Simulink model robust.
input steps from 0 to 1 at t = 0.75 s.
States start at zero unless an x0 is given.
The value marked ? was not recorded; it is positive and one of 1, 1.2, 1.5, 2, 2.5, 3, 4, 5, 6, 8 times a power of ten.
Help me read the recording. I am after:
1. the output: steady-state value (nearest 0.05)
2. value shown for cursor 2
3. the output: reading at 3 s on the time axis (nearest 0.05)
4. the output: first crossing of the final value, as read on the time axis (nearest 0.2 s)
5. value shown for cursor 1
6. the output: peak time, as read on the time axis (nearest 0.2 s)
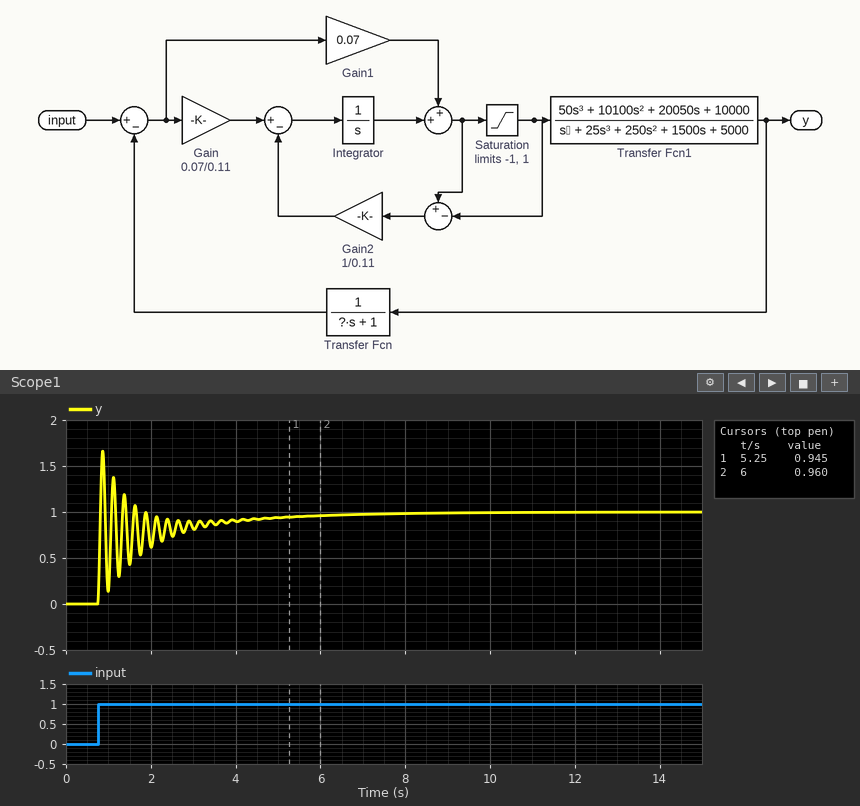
1.00
0.960
0.80
0.8 s
0.945
0.8 s
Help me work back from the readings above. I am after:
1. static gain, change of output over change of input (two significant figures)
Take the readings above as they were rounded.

1.0
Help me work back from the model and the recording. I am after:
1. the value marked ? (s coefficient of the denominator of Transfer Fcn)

0.025
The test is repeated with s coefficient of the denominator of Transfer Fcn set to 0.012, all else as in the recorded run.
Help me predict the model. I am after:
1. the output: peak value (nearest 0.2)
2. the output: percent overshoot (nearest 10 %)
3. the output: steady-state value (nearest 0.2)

1.4
40 %
1.0
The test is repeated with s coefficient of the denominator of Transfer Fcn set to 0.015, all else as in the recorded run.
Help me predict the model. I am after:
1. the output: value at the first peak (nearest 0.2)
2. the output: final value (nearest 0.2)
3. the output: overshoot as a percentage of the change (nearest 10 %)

1.4
1.0
50 %
